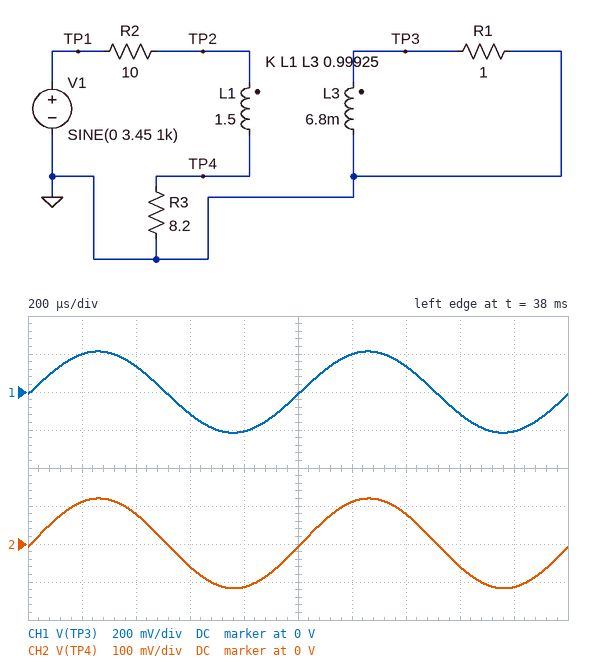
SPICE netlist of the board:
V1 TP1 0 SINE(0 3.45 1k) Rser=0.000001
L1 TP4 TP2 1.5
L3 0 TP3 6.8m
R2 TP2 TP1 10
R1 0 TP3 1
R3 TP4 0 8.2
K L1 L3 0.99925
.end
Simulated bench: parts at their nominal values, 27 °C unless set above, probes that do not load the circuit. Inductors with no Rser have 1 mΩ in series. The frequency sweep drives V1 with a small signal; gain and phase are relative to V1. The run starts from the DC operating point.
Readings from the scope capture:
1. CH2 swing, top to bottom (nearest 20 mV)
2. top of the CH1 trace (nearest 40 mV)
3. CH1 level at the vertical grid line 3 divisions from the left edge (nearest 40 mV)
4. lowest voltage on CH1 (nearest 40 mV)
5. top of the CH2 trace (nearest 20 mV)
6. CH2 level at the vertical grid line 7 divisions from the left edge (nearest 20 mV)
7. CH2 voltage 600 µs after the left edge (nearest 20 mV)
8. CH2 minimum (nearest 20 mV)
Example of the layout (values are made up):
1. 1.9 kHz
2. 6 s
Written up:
1. 240 mV
2. 200 mV
3. -120 mV
4. -200 mV
5. 120 mV
6. 80 mV
7. -60 mV
8. -120 mV
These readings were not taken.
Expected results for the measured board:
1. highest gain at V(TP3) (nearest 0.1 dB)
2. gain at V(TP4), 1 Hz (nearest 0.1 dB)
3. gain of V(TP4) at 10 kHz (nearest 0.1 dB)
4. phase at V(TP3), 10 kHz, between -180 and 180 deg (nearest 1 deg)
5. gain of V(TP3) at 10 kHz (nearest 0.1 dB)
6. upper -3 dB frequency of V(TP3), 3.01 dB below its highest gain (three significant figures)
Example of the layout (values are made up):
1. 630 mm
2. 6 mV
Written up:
1. -24.1 dB
2. -8.1 dB
3. -30.6 dB
4. -31 deg
5. -25.4 dB
6. 16.9 kHz
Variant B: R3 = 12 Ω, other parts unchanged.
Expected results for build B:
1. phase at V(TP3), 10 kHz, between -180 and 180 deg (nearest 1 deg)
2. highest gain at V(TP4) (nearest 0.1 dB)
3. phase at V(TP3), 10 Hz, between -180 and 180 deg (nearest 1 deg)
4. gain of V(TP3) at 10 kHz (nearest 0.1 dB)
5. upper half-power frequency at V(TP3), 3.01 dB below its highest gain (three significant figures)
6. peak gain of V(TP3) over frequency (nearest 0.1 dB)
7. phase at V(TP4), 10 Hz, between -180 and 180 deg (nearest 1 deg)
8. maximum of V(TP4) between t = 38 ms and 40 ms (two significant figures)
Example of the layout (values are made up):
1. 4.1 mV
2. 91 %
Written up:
1. -30 deg
2. -5.3 dB
3. 12 deg
4. -25.5 dB
5. 17.2 kHz
6. -24.3 dB
7. -55 deg
8. 170 mV
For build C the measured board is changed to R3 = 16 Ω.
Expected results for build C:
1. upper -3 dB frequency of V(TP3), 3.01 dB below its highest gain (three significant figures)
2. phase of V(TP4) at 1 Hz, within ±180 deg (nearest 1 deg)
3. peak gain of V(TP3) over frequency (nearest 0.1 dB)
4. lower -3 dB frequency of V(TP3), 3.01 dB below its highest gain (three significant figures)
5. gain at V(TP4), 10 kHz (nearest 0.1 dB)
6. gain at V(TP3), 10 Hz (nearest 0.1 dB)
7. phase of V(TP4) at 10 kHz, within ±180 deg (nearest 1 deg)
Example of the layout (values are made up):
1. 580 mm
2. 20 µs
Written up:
1. 17.5 kHz
2. -20 deg
3. -24.4 dB
4. 2.47 Hz
5. -25.0 dB
6. -24.7 dB
7. -30 deg
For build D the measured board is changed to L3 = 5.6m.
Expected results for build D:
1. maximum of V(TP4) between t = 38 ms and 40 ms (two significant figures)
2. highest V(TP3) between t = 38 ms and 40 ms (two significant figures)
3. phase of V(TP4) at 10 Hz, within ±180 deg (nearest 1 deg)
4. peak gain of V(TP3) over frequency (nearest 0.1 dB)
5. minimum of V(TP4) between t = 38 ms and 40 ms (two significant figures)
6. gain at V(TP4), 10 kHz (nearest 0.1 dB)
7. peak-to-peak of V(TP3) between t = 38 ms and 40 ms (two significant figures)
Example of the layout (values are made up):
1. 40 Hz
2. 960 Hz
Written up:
1. 100 mV
2. 200 mV
3. -60 deg
4. -24.9 dB
5. -97 mV
6. -31.8 dB
7. 390 mV
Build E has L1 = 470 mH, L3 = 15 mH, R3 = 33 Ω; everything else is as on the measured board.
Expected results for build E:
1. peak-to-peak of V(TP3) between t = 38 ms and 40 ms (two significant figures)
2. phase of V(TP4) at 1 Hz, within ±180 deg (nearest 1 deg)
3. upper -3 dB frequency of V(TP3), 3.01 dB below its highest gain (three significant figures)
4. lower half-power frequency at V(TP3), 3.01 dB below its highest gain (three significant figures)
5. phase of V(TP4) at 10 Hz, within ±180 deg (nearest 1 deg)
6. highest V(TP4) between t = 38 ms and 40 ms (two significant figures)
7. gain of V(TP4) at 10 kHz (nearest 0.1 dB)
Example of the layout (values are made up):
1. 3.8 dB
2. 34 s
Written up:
1. 520 mV
2. -4 deg
3. 16.8 kHz
4. 6.14 Hz
5. -15 deg
6. 1.5 V
7. -8.4 dB
